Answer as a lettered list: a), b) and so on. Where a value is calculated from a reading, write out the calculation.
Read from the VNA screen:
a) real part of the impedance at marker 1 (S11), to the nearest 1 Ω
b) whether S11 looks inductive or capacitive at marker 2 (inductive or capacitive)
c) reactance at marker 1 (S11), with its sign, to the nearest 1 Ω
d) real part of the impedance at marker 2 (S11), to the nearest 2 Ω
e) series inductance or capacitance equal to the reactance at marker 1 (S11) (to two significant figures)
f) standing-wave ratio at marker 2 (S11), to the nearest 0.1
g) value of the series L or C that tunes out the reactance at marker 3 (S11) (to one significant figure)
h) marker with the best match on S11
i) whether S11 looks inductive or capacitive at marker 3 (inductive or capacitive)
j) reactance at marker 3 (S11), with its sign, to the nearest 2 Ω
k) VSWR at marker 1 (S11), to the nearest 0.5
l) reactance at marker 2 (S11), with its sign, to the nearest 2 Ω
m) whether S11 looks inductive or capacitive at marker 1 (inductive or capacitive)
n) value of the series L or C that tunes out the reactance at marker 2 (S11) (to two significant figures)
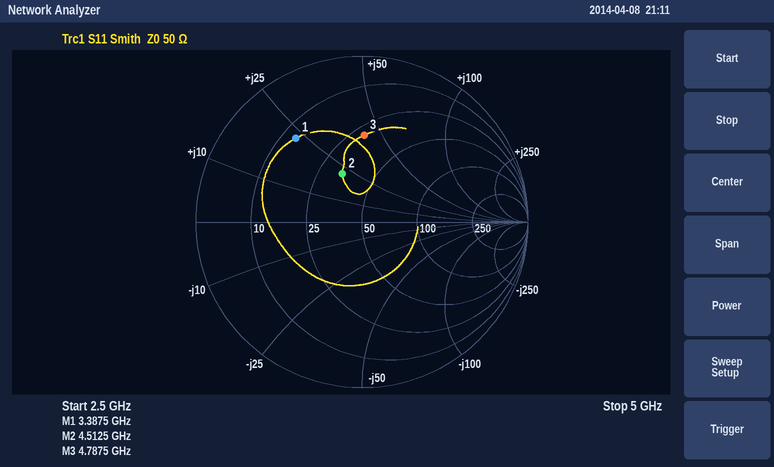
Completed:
a) 13 Ω
b) inductive
c) +23 Ω
d) 34 Ω
e) L = 23 Ω/(2π × 3.3875 GHz) ≈ 1.1 nH
f) 1.9
g) C = 1/(2π × 4.7875 GHz × 42 Ω) ≈ 792 fF, so 800 fF to one significant figure
h) marker 2
i) inductive
j) +42 Ω
k) 4.5
l) +22 Ω
m) inductive
n) C = 1/(2π × 4.5125 GHz × 22 Ω) ≈ 1.6 pF
